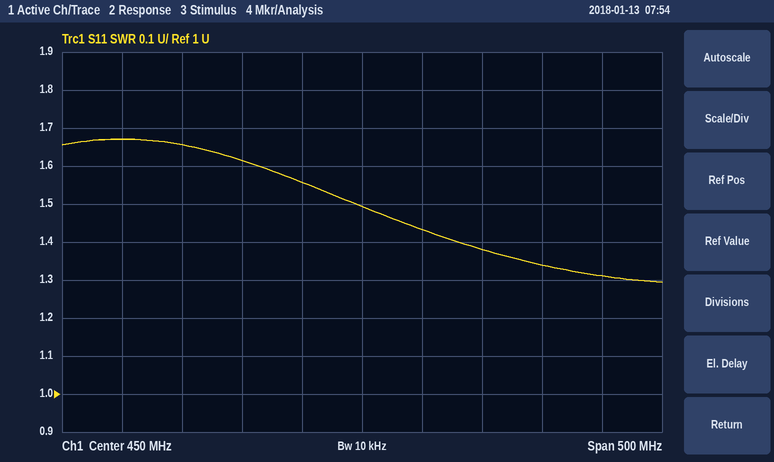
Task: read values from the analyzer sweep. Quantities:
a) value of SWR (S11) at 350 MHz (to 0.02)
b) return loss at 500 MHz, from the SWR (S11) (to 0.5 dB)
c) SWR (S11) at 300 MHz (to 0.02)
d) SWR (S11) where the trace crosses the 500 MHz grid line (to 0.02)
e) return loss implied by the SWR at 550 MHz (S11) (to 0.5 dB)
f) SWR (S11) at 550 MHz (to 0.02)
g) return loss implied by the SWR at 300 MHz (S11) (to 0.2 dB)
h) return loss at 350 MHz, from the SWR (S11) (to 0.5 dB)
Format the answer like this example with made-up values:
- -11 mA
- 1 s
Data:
- 1.62
- 15.0 dB
- 1.66
- 1.44
- 16.0 dB
- 1.38
- 12.2 dB
- 12.5 dB
